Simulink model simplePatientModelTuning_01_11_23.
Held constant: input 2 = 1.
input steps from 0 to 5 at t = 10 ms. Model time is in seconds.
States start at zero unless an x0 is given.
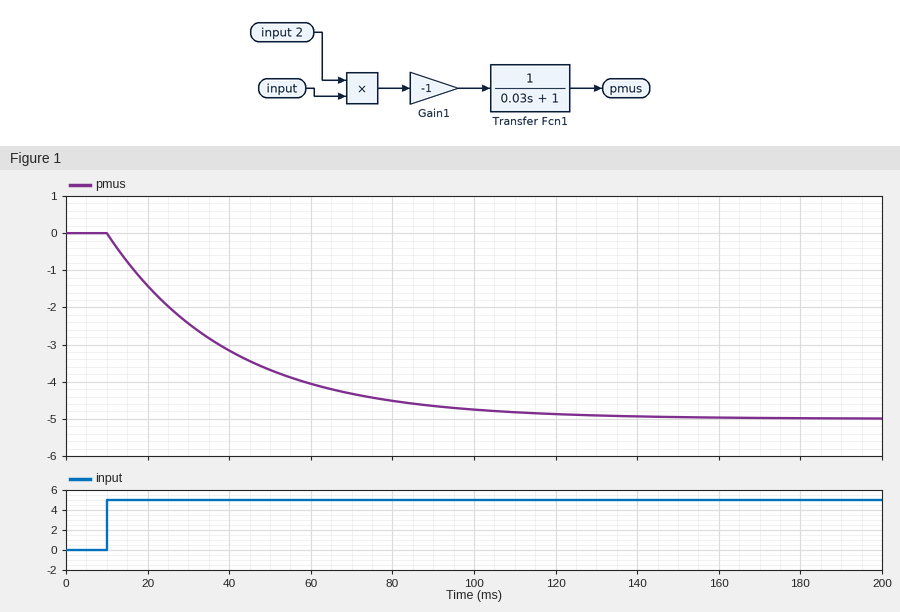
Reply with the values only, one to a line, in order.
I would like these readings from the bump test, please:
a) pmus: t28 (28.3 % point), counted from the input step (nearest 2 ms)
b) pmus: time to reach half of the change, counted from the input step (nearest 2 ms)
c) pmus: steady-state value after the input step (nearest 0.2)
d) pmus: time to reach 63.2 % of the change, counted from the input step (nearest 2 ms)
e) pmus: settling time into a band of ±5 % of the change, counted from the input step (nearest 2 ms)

10 ms
20 ms
-5.0
30 ms
90 ms
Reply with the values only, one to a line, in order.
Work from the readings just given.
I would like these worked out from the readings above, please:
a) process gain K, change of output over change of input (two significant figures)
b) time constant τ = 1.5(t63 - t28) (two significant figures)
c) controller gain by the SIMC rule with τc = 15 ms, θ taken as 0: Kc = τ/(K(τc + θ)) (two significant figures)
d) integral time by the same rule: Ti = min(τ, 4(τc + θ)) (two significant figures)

-1.0
30 ms
-2.0
30 ms
